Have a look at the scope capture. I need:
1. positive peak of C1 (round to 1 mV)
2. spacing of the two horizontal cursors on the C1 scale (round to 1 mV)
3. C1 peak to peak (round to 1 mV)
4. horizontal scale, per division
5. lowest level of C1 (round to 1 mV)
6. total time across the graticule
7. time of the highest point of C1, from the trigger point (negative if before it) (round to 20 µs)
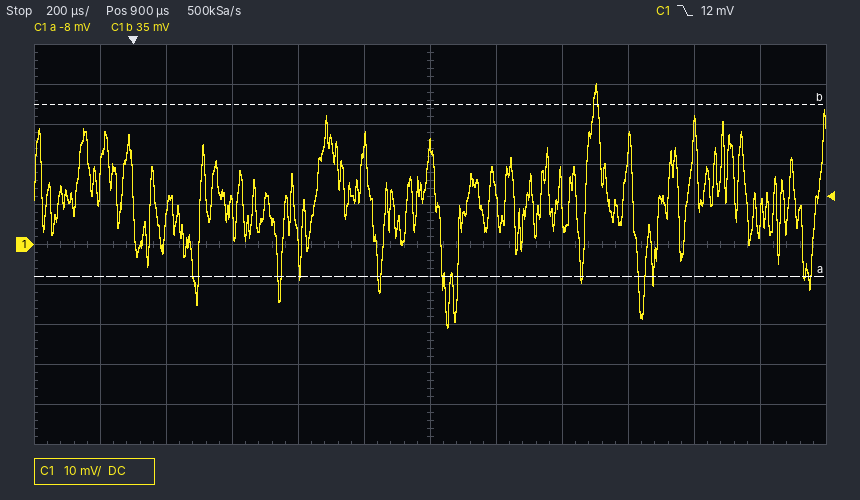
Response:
40 mV
43 mV
61 mV
200 µs
-21 mV
2.4 ms
+1.40 ms
